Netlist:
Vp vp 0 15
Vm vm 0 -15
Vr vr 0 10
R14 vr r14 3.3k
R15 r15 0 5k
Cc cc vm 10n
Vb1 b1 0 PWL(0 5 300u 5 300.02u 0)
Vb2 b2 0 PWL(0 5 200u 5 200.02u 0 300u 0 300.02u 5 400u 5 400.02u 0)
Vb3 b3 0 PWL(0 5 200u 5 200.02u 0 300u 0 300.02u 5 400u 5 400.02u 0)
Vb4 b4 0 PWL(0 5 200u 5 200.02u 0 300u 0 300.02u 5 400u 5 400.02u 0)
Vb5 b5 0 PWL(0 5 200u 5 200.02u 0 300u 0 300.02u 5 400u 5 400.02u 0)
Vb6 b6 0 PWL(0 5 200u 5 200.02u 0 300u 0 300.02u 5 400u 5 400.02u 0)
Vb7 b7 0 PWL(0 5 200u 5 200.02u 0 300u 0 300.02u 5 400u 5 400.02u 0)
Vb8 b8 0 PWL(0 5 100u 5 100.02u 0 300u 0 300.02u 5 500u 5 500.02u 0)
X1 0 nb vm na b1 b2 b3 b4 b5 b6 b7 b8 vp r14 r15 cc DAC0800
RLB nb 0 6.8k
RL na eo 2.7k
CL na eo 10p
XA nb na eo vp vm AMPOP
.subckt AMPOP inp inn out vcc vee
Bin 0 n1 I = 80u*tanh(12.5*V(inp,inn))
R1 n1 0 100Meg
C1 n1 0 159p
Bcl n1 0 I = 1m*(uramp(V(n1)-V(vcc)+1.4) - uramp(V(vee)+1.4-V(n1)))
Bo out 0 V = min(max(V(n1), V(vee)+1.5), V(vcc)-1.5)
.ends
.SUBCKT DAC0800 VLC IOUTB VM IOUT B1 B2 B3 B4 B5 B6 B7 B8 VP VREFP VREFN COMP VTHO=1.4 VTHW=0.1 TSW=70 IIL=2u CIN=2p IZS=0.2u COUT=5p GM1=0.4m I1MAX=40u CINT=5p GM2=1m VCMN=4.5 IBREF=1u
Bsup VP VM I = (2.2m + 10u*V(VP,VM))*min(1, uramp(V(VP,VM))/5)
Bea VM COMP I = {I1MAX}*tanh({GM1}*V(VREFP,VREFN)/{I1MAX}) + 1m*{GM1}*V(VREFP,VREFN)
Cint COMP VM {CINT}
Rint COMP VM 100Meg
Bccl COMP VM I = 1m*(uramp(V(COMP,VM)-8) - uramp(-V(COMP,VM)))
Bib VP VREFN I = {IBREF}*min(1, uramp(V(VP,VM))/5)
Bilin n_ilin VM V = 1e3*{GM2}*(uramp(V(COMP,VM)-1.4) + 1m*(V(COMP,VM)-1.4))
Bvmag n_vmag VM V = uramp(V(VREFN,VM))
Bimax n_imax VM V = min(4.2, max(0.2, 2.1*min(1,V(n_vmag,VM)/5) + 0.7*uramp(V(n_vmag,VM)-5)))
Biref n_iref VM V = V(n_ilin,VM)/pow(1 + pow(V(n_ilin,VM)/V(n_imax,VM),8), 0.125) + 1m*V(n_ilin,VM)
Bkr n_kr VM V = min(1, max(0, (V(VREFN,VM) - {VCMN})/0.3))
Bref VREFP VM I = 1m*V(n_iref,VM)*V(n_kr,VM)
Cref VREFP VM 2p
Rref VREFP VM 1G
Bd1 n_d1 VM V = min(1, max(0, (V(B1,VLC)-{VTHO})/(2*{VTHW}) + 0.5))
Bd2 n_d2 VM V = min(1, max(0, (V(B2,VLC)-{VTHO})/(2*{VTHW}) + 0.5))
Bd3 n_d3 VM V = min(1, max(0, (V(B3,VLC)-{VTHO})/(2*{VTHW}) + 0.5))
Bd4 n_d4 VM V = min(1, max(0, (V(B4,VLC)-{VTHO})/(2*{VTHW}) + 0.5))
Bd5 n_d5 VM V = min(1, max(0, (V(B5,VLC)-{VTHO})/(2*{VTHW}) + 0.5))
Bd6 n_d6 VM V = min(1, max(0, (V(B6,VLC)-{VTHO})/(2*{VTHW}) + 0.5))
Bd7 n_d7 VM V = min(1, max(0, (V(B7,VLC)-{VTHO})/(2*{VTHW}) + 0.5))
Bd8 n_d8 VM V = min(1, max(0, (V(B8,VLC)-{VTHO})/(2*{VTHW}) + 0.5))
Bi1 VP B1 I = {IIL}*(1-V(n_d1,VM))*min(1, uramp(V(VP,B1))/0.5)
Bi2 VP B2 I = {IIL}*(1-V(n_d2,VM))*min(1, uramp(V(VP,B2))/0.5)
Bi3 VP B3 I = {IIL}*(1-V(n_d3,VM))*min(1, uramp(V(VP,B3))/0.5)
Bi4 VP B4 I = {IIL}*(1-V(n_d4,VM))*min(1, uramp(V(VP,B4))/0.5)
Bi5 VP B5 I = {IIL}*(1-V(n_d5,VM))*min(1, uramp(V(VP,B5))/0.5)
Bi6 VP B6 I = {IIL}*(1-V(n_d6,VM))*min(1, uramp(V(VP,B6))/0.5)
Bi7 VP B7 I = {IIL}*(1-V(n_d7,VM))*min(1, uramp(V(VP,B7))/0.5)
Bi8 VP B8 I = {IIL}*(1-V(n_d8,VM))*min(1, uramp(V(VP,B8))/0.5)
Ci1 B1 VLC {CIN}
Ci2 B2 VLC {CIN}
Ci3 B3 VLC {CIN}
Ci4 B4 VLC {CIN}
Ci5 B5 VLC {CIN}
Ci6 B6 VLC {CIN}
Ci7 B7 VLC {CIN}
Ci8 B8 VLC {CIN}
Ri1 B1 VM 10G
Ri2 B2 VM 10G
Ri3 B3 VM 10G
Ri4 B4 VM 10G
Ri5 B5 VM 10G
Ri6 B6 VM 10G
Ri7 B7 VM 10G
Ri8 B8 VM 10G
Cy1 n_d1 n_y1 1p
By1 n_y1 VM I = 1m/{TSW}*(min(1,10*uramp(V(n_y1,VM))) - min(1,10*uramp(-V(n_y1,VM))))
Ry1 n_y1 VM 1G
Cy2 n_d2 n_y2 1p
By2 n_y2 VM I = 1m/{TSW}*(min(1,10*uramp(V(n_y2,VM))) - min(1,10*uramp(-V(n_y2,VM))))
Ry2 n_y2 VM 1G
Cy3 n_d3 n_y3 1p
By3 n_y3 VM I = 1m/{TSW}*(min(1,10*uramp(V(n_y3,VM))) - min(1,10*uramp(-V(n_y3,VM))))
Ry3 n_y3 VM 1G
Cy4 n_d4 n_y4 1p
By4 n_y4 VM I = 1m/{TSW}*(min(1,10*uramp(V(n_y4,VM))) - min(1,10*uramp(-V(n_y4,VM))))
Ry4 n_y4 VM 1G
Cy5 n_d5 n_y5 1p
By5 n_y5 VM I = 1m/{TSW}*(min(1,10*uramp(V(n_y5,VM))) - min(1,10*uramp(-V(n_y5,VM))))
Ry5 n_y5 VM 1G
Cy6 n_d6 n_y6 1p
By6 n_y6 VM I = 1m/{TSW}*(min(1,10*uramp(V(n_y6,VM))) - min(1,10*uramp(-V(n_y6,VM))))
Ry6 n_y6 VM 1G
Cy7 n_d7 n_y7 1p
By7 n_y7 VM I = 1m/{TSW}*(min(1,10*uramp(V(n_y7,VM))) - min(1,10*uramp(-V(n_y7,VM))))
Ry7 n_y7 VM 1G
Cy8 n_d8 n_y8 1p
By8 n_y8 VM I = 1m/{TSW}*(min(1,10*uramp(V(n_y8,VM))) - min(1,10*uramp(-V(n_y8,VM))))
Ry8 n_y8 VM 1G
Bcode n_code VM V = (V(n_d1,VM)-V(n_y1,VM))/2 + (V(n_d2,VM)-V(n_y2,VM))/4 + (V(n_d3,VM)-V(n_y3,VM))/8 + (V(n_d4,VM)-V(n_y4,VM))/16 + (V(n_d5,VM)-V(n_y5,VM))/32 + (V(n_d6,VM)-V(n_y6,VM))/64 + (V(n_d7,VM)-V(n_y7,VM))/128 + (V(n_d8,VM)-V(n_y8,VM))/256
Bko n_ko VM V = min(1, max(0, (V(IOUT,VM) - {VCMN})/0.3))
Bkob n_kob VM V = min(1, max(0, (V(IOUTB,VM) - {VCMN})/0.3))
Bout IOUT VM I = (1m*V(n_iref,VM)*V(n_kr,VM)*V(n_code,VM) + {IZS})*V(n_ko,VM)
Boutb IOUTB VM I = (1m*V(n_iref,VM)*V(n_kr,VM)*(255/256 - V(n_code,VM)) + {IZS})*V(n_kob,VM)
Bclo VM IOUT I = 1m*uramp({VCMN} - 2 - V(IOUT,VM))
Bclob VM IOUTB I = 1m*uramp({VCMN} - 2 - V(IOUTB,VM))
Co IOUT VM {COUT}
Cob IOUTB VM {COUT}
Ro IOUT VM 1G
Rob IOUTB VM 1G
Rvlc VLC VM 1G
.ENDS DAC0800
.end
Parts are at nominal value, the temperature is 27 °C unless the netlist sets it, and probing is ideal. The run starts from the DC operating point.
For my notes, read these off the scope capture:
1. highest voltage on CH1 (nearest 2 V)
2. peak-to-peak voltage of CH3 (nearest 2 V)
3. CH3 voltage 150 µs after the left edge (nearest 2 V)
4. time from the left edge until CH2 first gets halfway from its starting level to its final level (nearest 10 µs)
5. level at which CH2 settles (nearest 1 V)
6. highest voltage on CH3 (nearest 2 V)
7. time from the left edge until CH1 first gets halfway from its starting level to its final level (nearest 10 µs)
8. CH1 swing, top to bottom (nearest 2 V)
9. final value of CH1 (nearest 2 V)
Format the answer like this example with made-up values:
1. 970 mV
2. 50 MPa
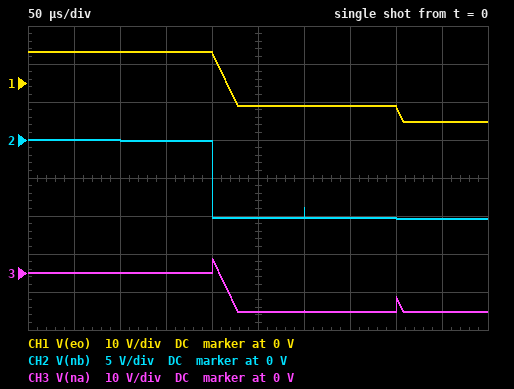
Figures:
1. 8 V
2. 14 V
3. 0 V
4. 200 µs
5. -10 V
6. 4 V
7. 220 µs
8. 18 V
9. -10 V
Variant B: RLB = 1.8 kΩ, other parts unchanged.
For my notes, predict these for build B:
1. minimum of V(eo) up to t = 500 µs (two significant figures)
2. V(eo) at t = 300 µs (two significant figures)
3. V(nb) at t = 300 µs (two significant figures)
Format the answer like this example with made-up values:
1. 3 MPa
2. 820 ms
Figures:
1. -5.4 V
2. 1.4 V
3. -2.7 V
